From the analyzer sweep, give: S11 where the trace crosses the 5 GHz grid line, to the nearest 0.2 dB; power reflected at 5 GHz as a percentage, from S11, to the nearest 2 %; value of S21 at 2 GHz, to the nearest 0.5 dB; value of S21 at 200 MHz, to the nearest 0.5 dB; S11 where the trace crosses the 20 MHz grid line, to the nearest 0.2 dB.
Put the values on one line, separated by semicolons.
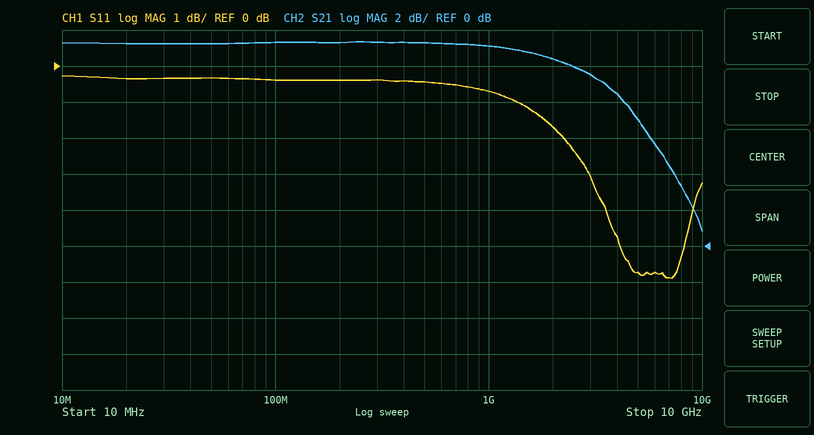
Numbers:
-5.8 dB; 26 %; 10.5 dB; 11.5 dB; -0.4 dB
